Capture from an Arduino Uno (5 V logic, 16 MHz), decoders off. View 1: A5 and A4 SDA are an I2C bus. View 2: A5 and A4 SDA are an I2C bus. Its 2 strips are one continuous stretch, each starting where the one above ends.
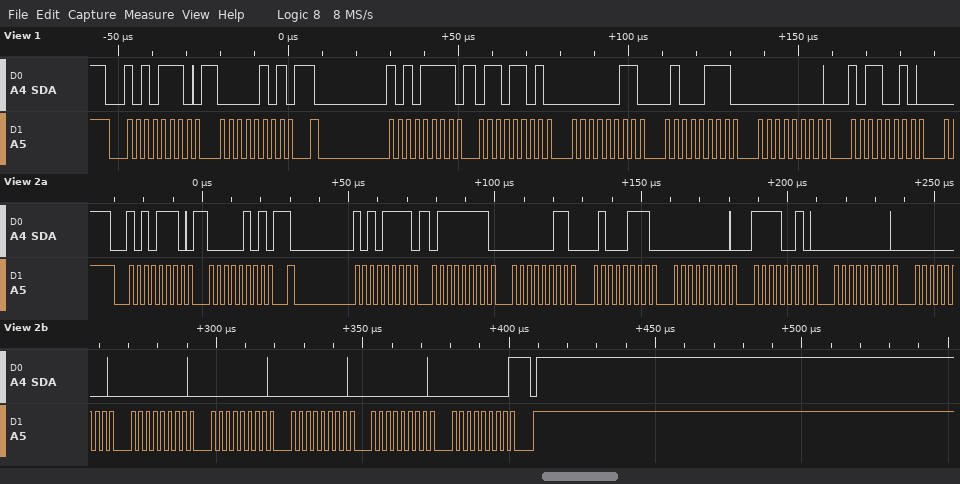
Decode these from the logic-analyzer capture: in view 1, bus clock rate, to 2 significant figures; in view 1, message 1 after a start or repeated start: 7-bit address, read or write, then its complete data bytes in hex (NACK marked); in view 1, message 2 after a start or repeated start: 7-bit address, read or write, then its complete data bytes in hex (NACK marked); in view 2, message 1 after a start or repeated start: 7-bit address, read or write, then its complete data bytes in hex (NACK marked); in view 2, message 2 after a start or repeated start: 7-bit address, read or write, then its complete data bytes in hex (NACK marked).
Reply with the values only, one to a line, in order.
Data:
400 kHz
0x57 write: 05
0x57 read: 6D 03 47 00 B2
0x57 write: 05
0x57 read: 7F 03 47 00 F2 00 00 00 00 00 00 00 NACK
